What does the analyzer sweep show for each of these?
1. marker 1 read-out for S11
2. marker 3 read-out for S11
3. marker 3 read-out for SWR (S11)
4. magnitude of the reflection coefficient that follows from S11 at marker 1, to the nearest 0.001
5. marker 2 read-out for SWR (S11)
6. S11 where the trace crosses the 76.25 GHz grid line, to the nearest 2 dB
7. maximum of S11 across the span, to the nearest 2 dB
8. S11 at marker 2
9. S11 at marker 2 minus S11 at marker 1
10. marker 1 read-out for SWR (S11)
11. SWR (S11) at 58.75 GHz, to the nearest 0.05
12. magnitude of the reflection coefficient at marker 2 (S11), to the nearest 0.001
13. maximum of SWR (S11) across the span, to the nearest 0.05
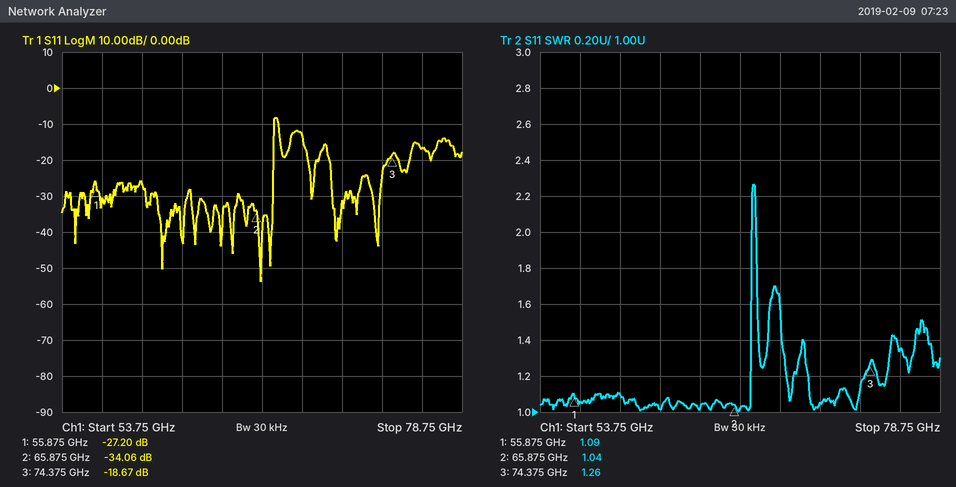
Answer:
-27.20 dB
-18.67 dB
1.26
0.044
1.04
-16 dB
-8 dB
-34.06 dB
-6.86 dB
1.09
1.10
0.020
2.25
